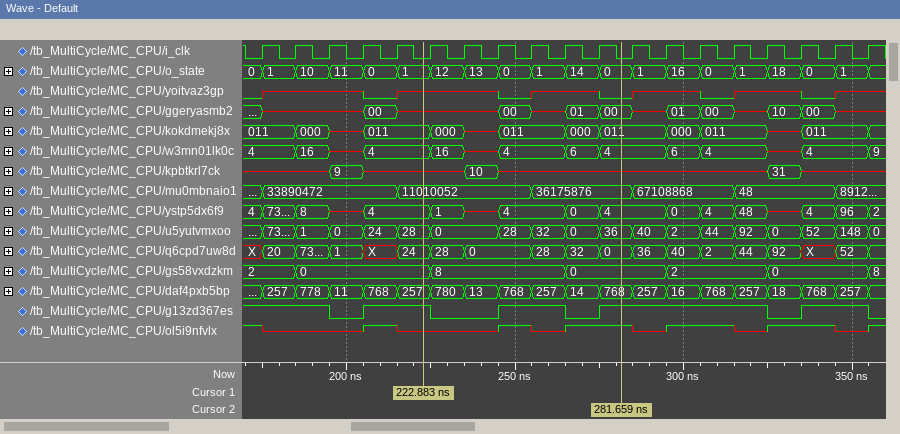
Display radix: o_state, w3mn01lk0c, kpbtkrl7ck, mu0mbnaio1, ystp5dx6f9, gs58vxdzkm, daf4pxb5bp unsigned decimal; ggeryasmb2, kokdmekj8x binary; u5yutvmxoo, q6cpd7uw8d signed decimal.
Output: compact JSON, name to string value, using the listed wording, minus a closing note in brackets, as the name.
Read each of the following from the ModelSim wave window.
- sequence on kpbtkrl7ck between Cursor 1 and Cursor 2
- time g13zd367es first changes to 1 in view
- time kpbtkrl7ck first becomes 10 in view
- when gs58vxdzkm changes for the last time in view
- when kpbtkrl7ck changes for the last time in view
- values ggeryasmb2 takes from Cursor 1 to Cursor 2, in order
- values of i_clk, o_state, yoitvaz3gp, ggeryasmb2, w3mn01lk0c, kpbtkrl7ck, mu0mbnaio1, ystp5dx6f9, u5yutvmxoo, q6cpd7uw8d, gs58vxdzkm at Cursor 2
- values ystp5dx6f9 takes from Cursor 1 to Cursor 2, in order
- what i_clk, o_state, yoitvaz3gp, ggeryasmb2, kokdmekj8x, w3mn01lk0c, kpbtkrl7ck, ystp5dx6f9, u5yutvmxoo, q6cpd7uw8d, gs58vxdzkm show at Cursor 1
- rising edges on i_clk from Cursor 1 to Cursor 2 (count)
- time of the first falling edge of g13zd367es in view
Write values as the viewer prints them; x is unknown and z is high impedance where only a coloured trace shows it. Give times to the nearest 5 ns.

{"sequence on kpbtkrl7ck between Cursor 1 and Cursor 2": "x, 10, x", "time g13zd367es first changes to 1 in view": "205 ns", "time kpbtkrl7ck first becomes 10 in view": "235 ns", "when gs58vxdzkm changes for the last time in view": "355 ns", "when kpbtkrl7ck changes for the last time in view": "335 ns", "values ggeryasmb2 takes from Cursor 1 to Cursor 2, in order": "x, 00, x, 01, 00", "values of i_clk, o_state, yoitvaz3gp, ggeryasmb2, w3mn01lk0c, kpbtkrl7ck, mu0mbnaio1, ystp5dx6f9, u5yutvmxoo, q6cpd7uw8d, gs58vxdzkm at Cursor 2": "i_clk=0, o_state=0, yoitvaz3gp=0, ggeryasmb2=00, w3mn01lk0c=4, kpbtkrl7ck=x, mu0mbnaio1=36175876, ystp5dx6f9=4, u5yutvmxoo=36, q6cpd7uw8d=0, gs58vxdzkm=0", "values ystp5dx6f9 takes from Cursor 1 to Cursor 2, in order": "4, 1, x, 4, 0, 4", "what i_clk, o_state, yoitvaz3gp, ggeryasmb2, kokdmekj8x, w3mn01lk0c, kpbtkrl7ck, ystp5dx6f9, u5yutvmxoo, q6cpd7uw8d, gs58vxdzkm show at Cursor 1": "i_clk=0, o_state=1, yoitvaz3gp=x, ggeryasmb2=x, kokdmekj8x=011, w3mn01lk0c=4, kpbtkrl7ck=x, ystp5dx6f9=4, u5yutvmxoo=28, q6cpd7uw8d=24, gs58vxdzkm=0", "rising edges on i_clk from Cursor 1 to Cursor 2": "6", "time of the first falling edge of g13zd367es in view": "195 ns"}
